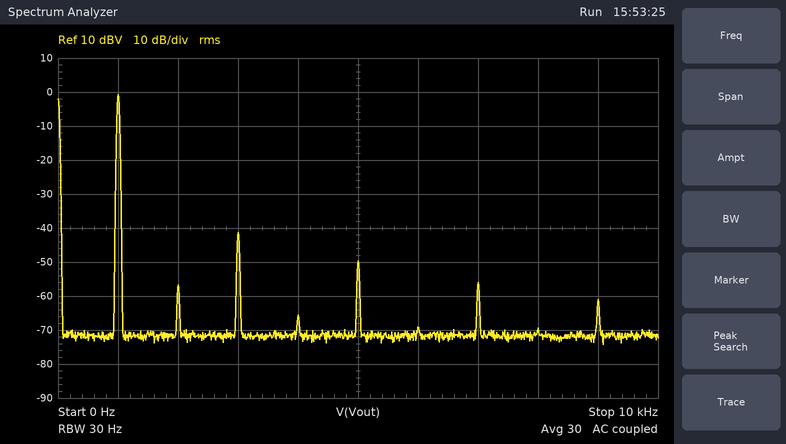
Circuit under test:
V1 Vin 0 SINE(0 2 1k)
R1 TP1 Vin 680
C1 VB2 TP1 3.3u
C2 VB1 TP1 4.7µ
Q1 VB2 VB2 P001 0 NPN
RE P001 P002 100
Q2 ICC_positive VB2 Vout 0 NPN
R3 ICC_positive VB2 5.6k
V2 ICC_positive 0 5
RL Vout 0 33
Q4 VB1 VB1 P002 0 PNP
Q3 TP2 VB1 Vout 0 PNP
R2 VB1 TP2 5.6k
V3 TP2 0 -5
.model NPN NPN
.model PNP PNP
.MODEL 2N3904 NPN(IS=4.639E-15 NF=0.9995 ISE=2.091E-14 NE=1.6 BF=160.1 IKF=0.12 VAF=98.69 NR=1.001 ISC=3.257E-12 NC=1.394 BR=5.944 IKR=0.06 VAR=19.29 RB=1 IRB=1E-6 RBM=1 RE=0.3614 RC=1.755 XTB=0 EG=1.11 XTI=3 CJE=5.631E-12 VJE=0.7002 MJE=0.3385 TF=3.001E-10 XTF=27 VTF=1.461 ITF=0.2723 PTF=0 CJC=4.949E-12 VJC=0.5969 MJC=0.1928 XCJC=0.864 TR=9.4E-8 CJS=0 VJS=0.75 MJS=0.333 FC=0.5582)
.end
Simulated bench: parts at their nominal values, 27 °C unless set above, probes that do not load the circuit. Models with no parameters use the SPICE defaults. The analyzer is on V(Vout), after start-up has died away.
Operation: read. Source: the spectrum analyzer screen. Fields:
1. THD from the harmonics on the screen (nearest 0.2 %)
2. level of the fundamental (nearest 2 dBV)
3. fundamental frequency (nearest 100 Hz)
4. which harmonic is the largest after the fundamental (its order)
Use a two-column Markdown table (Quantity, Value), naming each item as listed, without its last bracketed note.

| Quantity | Value |
|---|---|
| THD from the harmonics on the screen | 1.0 % |
| level of the fundamental | 0 dBV |
| fundamental frequency | 1.0 kHz |
| which harmonic is the largest after the fundamental | 3 |
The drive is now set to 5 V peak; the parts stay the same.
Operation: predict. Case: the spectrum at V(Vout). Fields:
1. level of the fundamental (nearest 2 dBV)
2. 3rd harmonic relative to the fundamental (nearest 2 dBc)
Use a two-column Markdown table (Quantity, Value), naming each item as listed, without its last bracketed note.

| Quantity | Value |
|---|---|
| level of the fundamental | 8 dBV |
| 3rd harmonic relative to the fundamental | -42 dBc |
